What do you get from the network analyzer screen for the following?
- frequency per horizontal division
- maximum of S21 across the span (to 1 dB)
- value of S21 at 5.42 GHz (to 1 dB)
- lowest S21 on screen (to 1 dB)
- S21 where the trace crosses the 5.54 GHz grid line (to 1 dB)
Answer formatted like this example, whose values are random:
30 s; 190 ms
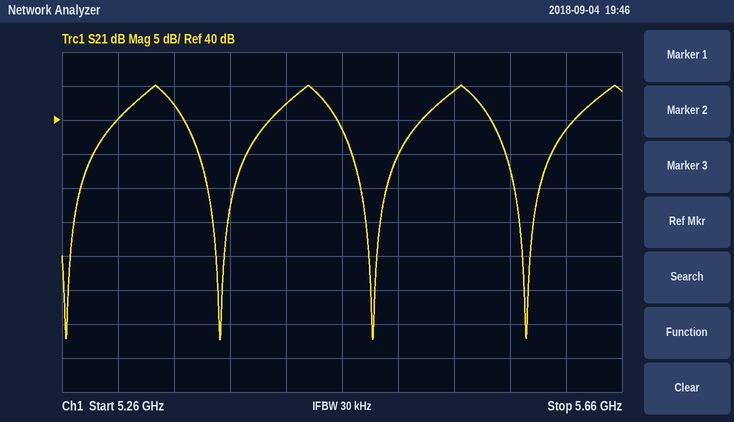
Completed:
40 MHz; 45 dB; 42 dB; 8 dB; 44 dB
